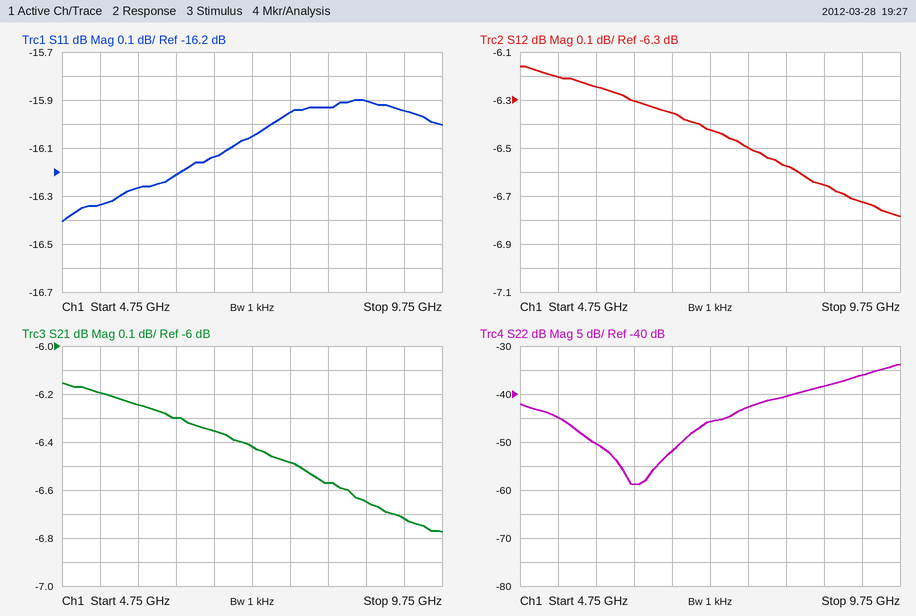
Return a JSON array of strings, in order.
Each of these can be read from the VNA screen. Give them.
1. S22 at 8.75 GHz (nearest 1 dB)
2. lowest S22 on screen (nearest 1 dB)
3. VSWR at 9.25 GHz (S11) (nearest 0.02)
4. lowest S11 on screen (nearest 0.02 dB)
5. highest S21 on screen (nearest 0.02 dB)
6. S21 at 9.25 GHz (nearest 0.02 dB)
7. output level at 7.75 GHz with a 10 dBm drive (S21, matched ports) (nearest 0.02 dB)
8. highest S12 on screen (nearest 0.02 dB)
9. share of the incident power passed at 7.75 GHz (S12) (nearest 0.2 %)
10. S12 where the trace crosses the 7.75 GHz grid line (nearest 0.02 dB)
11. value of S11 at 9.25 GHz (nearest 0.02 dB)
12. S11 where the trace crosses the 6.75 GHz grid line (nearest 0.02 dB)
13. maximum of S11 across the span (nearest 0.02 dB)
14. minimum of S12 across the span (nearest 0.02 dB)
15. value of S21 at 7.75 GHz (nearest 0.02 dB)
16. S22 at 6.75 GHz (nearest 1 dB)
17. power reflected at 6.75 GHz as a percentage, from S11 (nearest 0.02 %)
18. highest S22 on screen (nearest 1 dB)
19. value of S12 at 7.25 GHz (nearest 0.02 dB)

["-38 dB", "-59 dB", "1.38", "-16.40 dB", "-6.16 dB", "-6.72 dB", "3.52 dBm", "-6.16 dB", "22.4 %", "-6.50 dB", "-15.94 dB", "-16.14 dB", "-15.90 dB", "-6.78 dB", "-6.48 dB", "-52 dB", "2.44 %", "-34 dB", "-6.42 dB"]
